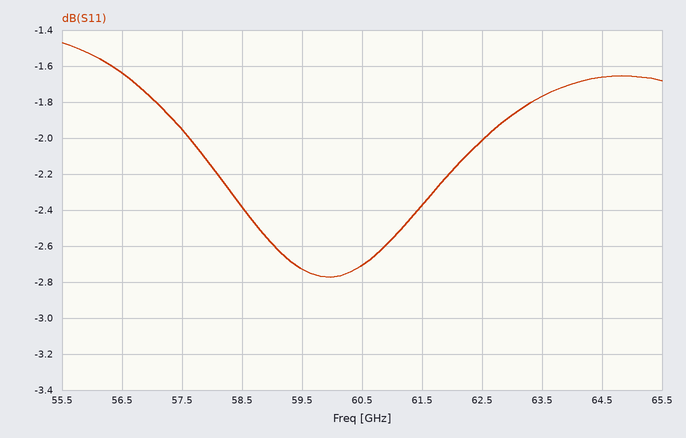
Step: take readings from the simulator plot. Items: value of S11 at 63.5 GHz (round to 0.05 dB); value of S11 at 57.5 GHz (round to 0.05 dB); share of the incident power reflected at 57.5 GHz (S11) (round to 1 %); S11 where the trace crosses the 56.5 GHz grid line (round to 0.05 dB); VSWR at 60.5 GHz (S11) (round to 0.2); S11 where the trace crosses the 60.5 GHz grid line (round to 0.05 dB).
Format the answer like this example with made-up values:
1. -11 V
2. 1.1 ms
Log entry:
1. -1.75 dB
2. -1.95 dB
3. 64 %
4. -1.65 dB
5. 6.4
6. -2.70 dB
